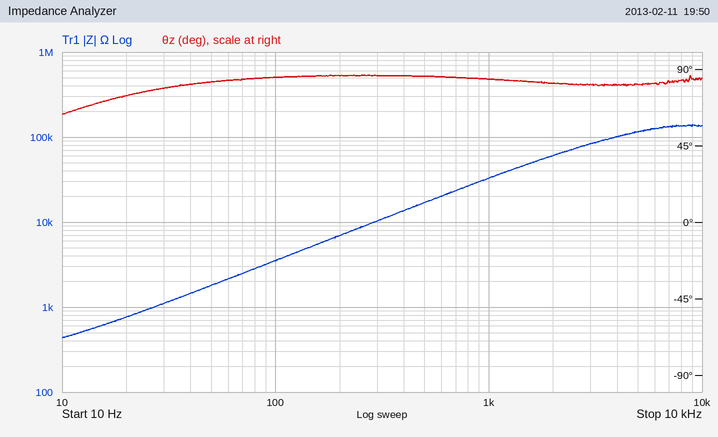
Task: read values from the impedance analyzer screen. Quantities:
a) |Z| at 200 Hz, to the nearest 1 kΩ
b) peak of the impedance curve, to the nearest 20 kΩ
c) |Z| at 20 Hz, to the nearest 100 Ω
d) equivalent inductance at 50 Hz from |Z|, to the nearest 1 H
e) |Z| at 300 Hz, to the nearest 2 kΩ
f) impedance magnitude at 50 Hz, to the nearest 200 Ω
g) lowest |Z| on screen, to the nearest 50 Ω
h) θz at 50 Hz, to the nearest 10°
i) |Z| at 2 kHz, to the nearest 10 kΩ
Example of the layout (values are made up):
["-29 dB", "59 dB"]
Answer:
["7 kΩ", "140 kΩ", "800 Ω", "6 H", "10 kΩ", "1.8 kΩ", "450 Ω", "80°", "60 kΩ"]
